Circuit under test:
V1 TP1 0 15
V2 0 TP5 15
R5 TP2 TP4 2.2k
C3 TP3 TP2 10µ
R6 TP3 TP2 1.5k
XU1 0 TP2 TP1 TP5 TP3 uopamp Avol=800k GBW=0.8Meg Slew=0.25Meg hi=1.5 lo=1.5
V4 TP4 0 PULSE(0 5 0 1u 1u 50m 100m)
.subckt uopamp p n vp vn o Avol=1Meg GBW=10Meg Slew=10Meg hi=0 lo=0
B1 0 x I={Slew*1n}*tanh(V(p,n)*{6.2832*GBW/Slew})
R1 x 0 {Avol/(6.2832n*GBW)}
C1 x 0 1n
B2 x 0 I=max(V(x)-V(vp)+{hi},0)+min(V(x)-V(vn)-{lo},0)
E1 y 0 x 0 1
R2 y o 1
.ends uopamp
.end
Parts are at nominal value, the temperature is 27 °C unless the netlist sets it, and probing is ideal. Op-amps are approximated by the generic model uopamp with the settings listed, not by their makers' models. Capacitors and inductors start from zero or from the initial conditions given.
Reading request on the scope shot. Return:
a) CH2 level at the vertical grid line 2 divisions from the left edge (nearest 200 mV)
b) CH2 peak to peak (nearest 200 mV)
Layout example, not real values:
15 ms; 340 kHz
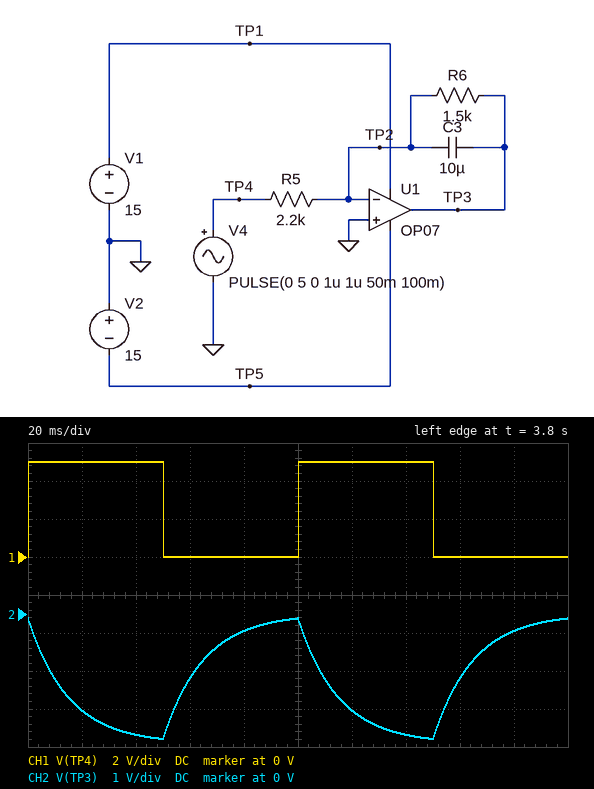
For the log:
-3.2 V; 3.2 V
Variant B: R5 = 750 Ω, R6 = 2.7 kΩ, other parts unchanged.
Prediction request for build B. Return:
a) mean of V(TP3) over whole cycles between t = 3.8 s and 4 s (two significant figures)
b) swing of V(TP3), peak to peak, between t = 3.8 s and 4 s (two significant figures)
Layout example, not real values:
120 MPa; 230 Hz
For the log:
-8.5 V; 11 V
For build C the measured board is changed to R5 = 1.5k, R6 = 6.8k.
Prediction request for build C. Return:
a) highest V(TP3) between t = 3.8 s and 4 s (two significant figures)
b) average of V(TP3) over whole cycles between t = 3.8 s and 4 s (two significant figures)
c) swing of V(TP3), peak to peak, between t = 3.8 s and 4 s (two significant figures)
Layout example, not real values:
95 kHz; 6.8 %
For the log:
-6.9 V; -11 V; 6.6 V
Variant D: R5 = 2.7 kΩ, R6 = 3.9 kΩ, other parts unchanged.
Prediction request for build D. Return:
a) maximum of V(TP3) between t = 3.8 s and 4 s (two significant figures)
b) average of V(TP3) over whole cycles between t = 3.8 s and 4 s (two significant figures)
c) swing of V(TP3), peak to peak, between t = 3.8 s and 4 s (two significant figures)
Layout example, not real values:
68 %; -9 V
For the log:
-1.6 V; -3.6 V; 4.1 V
